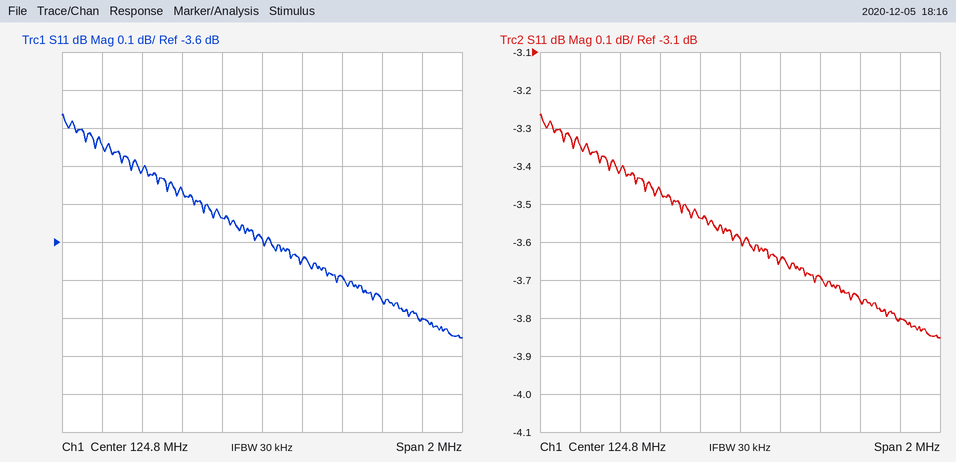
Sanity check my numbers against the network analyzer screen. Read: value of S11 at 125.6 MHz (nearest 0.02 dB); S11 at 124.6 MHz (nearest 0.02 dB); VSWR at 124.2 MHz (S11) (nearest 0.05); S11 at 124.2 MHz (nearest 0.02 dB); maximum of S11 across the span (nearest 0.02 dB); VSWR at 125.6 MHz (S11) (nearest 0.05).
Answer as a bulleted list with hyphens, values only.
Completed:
- -3.80 dB
- -3.54 dB
- 5.15
- -3.42 dB
- -3.26 dB
- 4.65
